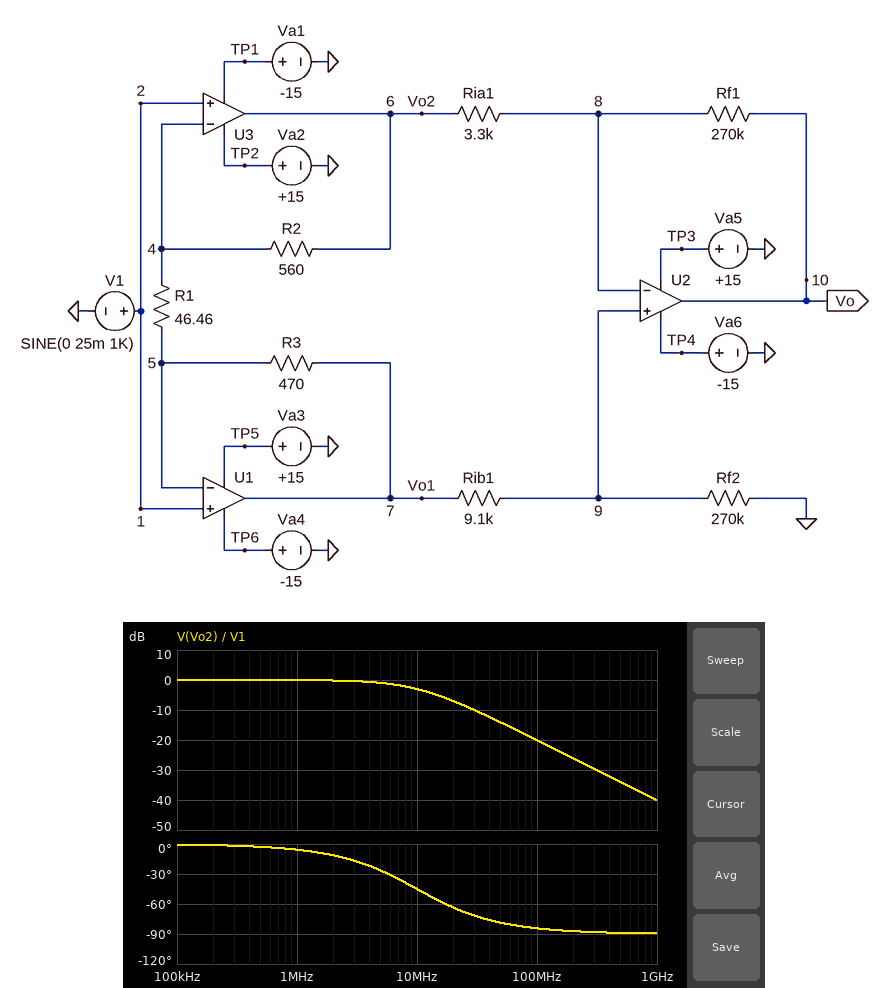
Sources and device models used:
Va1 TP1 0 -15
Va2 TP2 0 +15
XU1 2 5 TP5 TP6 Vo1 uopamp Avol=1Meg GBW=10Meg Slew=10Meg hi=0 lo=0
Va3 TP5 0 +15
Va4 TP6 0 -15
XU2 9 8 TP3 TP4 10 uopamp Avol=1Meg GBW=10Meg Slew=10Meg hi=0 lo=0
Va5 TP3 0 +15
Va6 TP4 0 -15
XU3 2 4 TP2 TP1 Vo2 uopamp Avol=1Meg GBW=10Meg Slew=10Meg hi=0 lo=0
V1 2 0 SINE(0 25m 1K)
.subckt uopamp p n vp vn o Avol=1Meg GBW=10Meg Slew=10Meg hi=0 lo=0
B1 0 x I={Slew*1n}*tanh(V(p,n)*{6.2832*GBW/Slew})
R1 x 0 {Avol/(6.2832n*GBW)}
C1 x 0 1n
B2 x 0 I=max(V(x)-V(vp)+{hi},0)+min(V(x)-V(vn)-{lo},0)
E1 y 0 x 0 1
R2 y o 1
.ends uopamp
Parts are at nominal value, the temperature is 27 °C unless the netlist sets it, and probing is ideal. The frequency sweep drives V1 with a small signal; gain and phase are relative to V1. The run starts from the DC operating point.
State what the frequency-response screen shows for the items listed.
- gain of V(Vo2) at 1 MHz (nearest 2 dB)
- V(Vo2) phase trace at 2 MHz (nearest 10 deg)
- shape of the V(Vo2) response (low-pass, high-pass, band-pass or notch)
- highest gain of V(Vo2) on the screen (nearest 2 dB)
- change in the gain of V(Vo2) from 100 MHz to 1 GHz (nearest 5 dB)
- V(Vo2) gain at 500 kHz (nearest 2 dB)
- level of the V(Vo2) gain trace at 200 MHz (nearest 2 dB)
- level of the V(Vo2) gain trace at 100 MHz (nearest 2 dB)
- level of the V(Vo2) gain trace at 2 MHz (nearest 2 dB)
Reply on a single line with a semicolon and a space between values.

0 dB; -10 deg; low-pass; 0 dB; -20 dB; 0 dB; -26 dB; -20 dB; 0 dB
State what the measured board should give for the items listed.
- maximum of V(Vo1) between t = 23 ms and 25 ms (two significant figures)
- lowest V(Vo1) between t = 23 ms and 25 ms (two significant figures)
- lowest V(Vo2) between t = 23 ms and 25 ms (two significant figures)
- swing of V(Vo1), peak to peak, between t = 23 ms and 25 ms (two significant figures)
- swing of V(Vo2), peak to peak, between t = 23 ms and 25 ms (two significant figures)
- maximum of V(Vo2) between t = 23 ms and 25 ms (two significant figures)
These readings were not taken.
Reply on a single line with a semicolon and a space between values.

25 mV; -25 mV; -25 mV; 50 mV; 50 mV; 25 mV
